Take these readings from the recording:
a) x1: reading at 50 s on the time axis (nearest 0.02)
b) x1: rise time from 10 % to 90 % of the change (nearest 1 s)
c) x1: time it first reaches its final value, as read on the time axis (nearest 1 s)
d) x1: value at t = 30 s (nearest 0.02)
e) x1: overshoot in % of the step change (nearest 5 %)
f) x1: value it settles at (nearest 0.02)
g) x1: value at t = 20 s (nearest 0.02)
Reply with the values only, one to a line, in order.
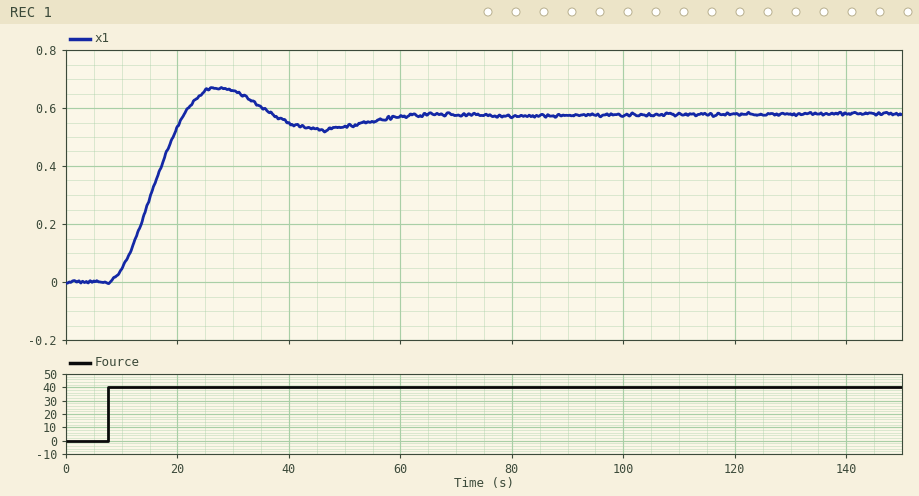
0.54
9 s
21 s
0.66
15 %
0.58
0.54
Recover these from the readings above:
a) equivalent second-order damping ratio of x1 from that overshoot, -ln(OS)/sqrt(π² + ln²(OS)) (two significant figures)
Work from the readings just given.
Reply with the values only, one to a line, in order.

0.52
